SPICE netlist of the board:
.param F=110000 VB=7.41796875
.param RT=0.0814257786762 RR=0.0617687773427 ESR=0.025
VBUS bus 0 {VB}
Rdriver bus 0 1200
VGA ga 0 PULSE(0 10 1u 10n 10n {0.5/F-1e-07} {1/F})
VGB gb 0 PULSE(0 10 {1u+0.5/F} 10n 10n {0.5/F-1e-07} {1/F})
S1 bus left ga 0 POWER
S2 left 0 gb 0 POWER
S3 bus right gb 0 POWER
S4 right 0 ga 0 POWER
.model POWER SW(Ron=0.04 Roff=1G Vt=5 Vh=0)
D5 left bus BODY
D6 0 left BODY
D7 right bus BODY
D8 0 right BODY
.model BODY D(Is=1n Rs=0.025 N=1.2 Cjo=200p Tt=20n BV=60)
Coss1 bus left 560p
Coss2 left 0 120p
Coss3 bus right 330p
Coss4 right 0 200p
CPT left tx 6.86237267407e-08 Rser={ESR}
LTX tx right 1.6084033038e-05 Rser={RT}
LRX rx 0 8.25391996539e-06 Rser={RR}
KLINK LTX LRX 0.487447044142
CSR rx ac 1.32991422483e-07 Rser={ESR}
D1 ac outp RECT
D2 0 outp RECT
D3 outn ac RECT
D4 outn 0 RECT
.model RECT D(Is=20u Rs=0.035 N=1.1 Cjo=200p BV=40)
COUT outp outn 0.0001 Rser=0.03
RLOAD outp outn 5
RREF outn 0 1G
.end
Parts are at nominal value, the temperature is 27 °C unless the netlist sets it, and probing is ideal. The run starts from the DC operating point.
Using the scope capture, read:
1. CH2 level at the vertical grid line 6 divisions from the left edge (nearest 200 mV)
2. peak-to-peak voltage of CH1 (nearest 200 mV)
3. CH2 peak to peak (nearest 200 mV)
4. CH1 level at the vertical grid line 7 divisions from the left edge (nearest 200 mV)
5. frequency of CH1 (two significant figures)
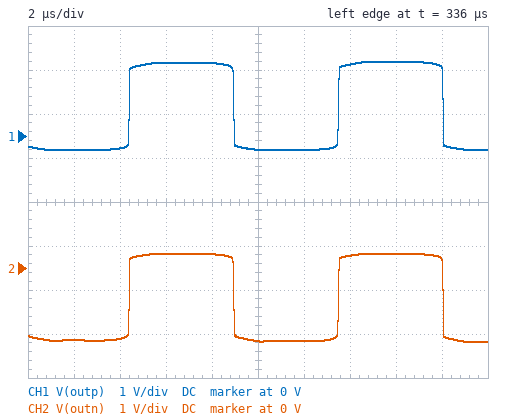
-1.6 V
2.0 V
2.0 V
1.6 V
110 kHz
